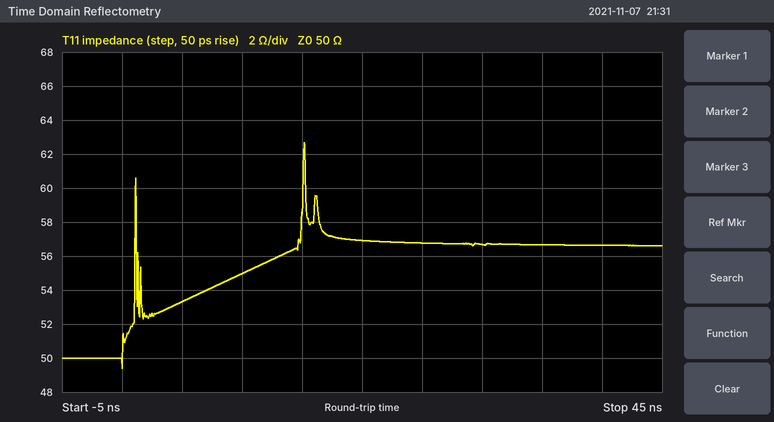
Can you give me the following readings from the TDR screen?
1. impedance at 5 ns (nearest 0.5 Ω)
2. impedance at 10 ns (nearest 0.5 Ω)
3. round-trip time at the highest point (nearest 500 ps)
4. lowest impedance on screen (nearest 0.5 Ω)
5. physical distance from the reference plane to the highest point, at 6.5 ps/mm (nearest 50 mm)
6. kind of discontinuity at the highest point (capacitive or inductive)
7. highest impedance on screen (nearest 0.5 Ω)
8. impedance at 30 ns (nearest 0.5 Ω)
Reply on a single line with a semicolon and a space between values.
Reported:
53.5 Ω; 55.0 Ω; 15.0 ns; 49.5 Ω; 1.15 m; inductive; 62.5 Ω; 56.5 Ω
